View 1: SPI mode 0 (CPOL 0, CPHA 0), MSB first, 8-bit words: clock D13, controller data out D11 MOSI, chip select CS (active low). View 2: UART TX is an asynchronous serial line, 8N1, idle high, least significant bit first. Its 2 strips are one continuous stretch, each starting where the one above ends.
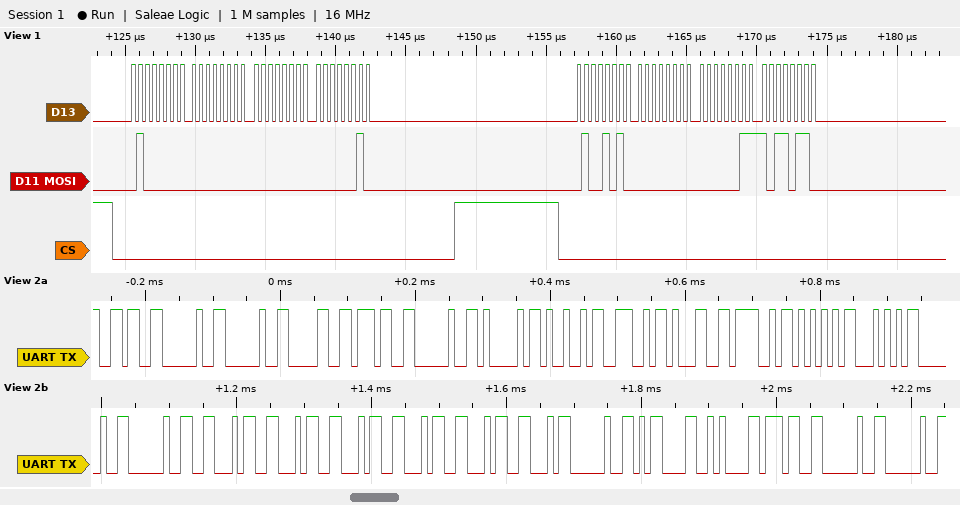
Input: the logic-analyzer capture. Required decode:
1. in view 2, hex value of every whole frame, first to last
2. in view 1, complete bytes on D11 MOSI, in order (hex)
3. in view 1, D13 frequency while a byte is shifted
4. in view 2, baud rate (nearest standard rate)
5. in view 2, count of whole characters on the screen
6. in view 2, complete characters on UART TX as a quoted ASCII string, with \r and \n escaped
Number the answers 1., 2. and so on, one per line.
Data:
1. 36 20 20 30 37 20 41 49 4E 31 4F 55 54 20 20 46 46 46 46 46 46 20 0D 0A 37 20 20
2. 40 00 00 02 4A 00 03 B6
3. 2 MHz
4. 115200 baud
5. 27
6. "6  07 AIN1OUT  FFFFFF \r\n7  "
